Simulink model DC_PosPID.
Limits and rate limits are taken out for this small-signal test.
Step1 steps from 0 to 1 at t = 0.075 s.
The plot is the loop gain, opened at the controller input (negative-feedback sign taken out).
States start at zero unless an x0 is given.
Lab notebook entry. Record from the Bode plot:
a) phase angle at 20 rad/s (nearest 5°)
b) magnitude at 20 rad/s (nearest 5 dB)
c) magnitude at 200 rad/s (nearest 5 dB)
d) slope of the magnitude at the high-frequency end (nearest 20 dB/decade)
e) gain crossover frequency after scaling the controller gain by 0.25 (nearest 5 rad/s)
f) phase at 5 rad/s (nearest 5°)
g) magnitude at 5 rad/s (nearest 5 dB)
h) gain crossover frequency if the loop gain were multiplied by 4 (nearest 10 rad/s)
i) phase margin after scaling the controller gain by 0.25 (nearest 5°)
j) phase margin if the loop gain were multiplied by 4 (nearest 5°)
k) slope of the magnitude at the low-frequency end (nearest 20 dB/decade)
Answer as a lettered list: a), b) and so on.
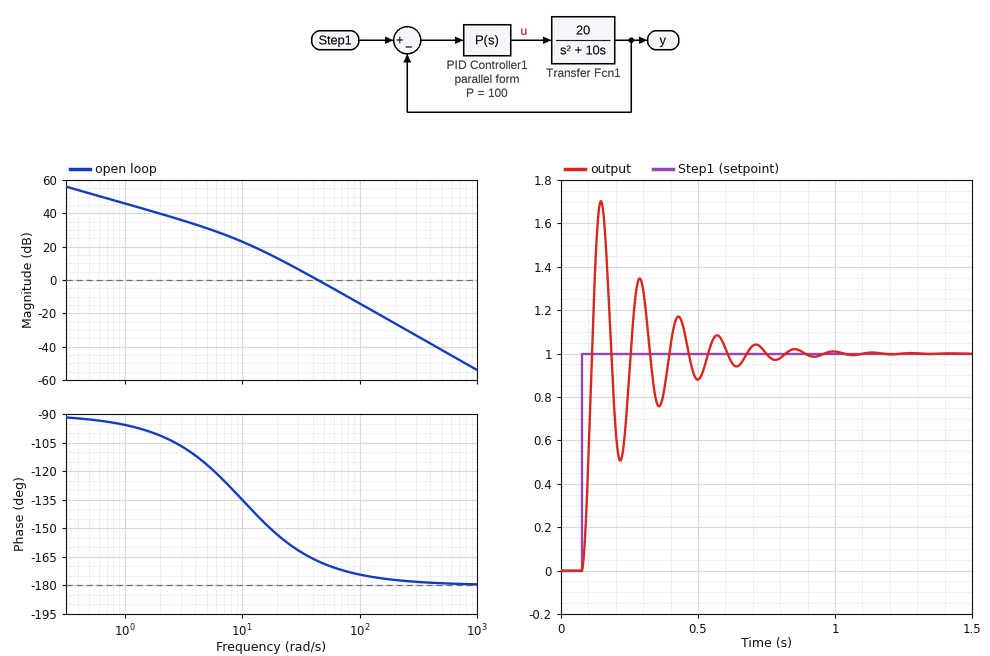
a) -155°
b) 15 dB
c) -25 dB
d) -40 dB/decade
e) 20 rad/s
f) -115°
g) 30 dB
h) 90 rad/s
i) 25°
j) 5°
k) -20 dB/decade
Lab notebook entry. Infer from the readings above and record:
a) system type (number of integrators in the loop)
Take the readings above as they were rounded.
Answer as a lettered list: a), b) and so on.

a) 1
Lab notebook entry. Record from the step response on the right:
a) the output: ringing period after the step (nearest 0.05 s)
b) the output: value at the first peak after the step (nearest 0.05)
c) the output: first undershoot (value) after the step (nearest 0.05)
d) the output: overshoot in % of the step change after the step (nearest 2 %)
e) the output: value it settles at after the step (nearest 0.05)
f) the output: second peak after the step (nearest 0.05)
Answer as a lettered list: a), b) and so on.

a) 0.15 s
b) 1.70
c) 0.50
d) 70 %
e) 1.00
f) 1.35
